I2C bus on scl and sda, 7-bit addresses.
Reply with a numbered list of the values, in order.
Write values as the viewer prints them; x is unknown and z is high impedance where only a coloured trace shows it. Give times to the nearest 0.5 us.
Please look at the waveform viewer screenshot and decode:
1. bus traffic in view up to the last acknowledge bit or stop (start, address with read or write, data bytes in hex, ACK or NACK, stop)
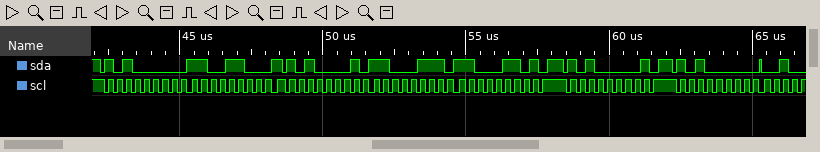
1. start, address 50 write ACK, CC ACK, repeated start, address 50 read ACK, C7 ACK, C6 NACK, stop, start, address 50 write NACK, stop, start, address 50 write ACK
